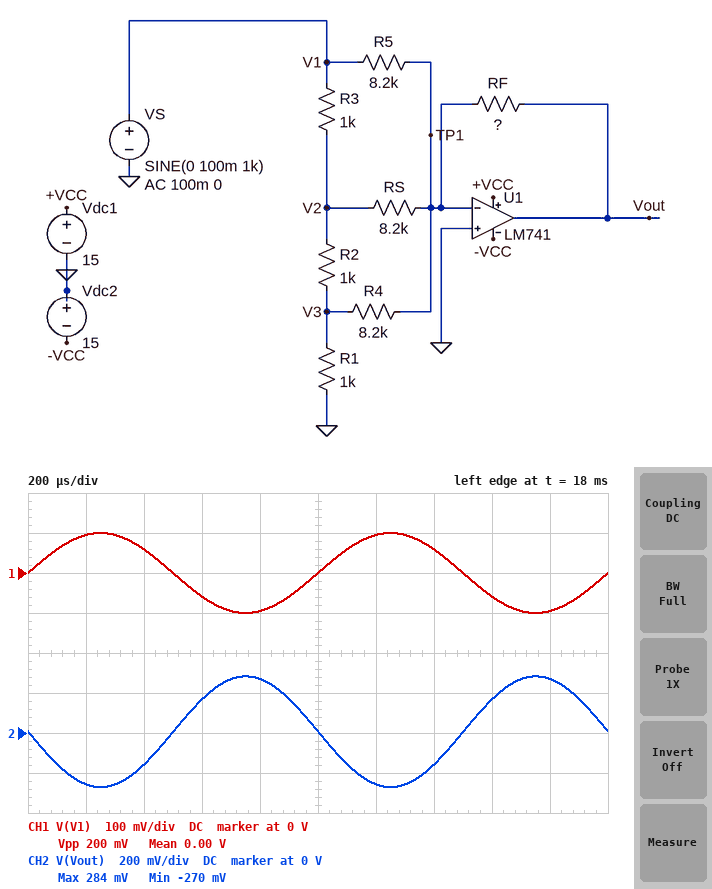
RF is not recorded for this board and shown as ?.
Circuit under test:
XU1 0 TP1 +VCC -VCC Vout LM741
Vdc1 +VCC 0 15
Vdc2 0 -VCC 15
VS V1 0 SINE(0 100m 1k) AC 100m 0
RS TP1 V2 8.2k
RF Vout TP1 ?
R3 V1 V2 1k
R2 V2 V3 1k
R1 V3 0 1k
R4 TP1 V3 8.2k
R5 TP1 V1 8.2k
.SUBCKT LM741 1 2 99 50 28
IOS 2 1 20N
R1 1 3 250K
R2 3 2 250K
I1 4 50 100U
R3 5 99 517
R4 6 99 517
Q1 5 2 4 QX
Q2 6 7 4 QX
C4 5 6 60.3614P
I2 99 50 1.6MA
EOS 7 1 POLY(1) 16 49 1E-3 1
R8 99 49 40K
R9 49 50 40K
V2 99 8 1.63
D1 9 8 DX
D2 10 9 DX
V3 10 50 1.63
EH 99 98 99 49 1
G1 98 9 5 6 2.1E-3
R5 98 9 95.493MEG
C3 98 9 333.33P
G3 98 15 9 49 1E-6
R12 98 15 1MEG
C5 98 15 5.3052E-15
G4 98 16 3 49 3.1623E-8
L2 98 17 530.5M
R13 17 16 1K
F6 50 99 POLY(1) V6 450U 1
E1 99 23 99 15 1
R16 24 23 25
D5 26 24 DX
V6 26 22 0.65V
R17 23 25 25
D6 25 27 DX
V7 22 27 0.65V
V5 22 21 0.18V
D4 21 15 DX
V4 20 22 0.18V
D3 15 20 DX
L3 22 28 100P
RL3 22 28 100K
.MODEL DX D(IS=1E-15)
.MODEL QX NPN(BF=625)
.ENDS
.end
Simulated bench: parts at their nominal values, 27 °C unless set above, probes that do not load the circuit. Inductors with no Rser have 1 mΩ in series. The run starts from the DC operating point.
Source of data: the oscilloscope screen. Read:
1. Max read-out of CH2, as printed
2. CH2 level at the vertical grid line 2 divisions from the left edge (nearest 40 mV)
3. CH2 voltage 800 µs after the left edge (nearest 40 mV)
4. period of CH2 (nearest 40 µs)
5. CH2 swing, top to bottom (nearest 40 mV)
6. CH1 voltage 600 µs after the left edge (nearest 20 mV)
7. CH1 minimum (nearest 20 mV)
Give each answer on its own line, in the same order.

284 mV
-160 mV
280 mV
1.00 ms
560 mV
-60 mV
-100 mV
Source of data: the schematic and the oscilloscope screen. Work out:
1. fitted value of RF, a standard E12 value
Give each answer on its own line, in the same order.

12 kΩ
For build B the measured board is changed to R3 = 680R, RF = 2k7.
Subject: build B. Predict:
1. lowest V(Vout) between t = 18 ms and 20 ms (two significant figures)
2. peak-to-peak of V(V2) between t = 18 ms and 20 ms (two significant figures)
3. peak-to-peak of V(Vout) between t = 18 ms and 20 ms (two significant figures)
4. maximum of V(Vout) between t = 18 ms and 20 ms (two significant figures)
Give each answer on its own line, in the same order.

-64 mV
140 mV
130 mV
69 mV
